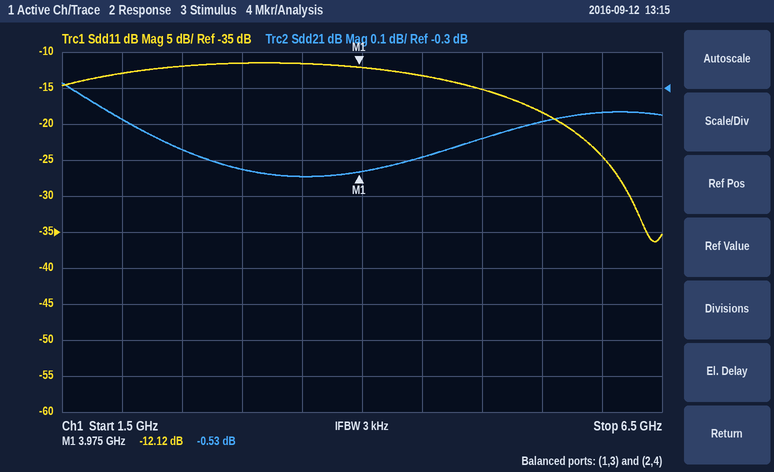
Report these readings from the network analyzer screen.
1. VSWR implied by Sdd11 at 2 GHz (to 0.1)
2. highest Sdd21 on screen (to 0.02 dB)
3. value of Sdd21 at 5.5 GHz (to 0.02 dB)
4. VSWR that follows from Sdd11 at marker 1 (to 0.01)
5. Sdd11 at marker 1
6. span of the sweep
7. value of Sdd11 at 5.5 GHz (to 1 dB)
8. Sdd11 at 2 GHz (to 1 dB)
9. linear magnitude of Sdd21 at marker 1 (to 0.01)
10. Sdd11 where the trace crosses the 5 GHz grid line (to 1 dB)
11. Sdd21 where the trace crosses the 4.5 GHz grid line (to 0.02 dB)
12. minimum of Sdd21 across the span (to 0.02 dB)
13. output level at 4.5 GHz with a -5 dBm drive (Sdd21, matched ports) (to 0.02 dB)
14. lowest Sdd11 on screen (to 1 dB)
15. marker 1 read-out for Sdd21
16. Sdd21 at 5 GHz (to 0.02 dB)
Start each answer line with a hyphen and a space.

- 1.6
- -0.28 dB
- -0.40 dB
- 1.66
- -12.12 dB
- 5 GHz
- -18 dB
- -13 dB
- 0.94
- -15 dB
- -0.50 dB
- -0.54 dB
- -5.50 dBm
- -36 dB
- -0.53 dB
- -0.44 dB
